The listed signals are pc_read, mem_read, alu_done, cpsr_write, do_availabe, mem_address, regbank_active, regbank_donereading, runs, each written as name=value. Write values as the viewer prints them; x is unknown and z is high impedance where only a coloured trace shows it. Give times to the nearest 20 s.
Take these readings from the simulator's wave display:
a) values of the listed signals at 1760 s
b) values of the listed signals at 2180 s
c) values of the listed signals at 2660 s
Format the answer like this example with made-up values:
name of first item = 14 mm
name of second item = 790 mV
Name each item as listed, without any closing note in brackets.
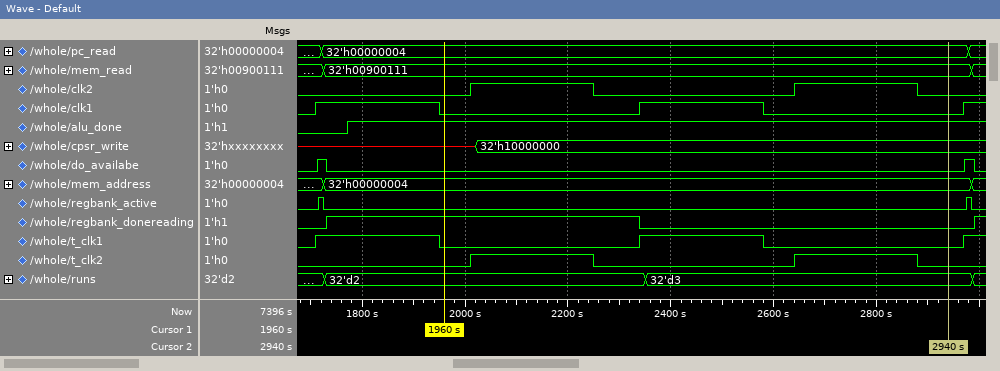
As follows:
values of the listed signals at 1760 s = pc_read=32'h00000004, mem_read=32'h00900111, alu_done=0, cpsr_write=x, do_availabe=0, mem_address=32'h00000004, regbank_active=0, regbank_donereading=1, runs=32'd2
values of the listed signals at 2180 s = pc_read=32'h00000004, mem_read=32'h00900111, alu_done=1, cpsr_write=32'h10000000, do_availabe=0, mem_address=32'h00000004, regbank_active=0, regbank_donereading=1, runs=32'd2
values of the listed signals at 2660 s = pc_read=32'h00000004, mem_read=32'h00900111, alu_done=1, cpsr_write=32'h10000000, do_availabe=0, mem_address=32'h00000004, regbank_active=0, regbank_donereading=0, runs=32'd3
